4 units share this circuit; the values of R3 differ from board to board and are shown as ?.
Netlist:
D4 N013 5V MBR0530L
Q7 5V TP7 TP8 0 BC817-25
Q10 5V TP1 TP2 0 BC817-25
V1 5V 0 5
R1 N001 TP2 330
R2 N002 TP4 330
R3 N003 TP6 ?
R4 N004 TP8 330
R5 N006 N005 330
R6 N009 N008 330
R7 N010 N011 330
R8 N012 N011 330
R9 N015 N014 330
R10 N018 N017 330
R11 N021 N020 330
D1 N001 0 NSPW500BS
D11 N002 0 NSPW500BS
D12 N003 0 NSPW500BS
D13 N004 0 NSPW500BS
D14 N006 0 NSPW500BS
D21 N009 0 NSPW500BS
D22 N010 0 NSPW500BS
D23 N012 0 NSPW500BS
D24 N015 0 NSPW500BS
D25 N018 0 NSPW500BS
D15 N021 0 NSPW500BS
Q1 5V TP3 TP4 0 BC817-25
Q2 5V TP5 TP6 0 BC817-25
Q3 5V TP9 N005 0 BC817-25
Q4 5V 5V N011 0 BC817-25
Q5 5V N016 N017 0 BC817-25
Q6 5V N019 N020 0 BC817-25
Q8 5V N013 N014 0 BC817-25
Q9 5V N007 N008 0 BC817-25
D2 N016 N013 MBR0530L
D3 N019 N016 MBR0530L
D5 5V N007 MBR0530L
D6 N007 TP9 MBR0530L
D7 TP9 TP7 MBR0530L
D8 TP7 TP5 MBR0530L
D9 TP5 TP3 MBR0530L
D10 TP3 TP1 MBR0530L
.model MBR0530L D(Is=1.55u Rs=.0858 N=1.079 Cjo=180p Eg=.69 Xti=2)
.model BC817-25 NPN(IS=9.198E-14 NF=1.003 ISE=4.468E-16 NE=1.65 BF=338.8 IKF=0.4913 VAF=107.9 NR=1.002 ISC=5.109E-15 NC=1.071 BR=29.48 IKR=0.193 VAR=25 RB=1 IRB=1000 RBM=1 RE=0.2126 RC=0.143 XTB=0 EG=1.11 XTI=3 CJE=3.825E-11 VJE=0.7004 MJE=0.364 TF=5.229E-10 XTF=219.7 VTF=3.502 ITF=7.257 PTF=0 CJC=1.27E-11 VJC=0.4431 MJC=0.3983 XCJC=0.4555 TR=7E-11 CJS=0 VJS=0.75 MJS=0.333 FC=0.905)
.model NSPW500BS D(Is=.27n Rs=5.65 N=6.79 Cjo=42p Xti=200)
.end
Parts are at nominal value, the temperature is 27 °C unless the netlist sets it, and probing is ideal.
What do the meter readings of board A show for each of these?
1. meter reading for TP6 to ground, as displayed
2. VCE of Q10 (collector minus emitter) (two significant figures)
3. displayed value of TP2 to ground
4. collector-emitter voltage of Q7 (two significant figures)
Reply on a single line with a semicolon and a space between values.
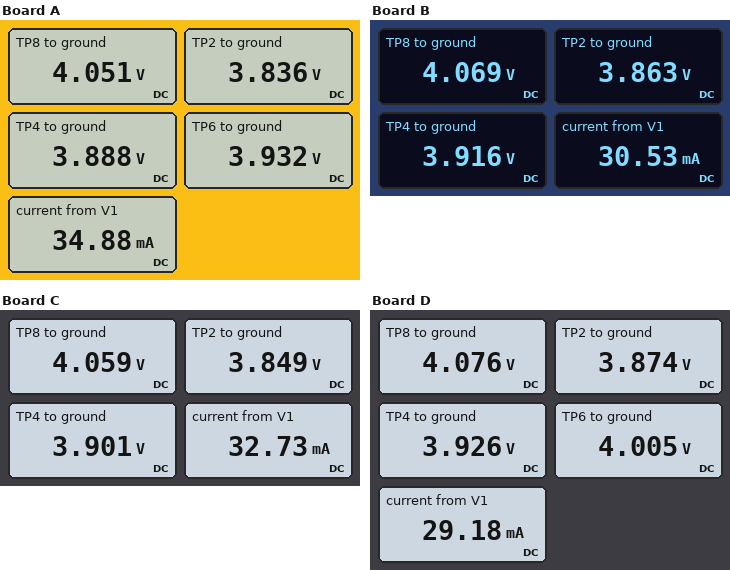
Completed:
3.932 V; 1.2 V; 3.836 V; 950 mV
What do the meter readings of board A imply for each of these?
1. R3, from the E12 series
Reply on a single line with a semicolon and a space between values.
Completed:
100 Ω
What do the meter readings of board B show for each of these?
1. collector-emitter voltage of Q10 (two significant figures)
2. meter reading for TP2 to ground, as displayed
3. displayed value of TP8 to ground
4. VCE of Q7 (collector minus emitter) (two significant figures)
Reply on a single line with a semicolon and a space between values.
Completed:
1.1 V; 3.863 V; 4.069 V; 930 mV
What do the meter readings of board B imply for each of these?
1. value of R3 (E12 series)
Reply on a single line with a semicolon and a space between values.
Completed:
270 Ω
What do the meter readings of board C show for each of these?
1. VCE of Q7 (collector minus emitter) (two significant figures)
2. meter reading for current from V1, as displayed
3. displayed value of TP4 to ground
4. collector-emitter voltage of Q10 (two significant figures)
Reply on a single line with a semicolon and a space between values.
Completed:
940 mV; 32.73 mA; 3.901 V; 1.2 V
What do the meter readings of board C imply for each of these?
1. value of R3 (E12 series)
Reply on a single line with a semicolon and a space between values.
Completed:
150 Ω
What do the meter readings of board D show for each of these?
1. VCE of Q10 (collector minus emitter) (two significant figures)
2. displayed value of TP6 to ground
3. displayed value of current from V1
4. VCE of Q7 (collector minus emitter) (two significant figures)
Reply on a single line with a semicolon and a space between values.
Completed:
1.1 V; 4.005 V; 29.18 mA; 920 mV
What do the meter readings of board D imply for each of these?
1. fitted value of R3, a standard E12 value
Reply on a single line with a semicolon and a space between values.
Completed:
470 Ω
